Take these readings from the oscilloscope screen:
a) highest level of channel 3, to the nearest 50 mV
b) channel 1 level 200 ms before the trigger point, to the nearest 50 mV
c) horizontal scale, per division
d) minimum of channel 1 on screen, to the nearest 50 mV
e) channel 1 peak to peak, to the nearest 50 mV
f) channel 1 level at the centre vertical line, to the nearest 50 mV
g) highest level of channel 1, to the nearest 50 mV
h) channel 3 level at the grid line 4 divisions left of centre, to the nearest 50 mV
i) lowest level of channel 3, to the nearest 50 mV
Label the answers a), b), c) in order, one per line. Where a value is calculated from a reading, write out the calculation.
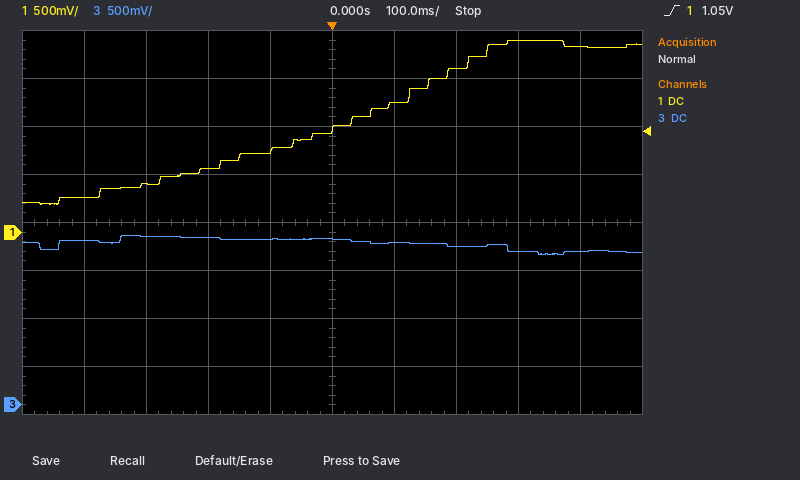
a) 1.75 V
b) 650 mV
c) 100 ms
d) 300 mV
e) 2.00 V − (300 mV) = 1.70 V
f) 1.05 V
g) 2.00 V
h) 1.70 V
i) 1.55 V
